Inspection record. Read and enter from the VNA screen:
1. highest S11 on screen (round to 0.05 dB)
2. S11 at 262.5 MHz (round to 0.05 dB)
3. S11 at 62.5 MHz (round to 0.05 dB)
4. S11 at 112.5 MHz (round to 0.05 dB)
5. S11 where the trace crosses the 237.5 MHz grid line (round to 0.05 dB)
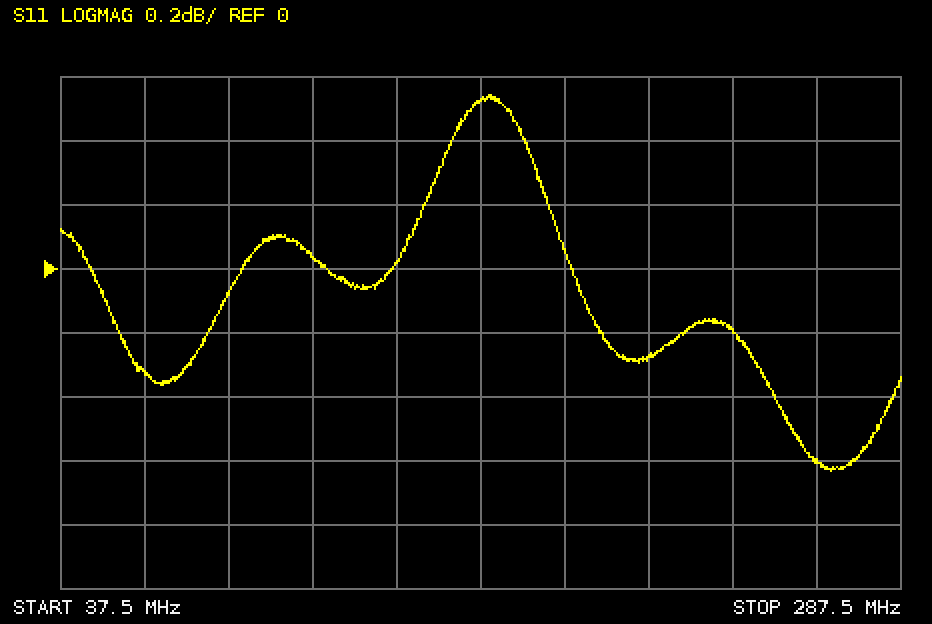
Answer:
0.55 dB
-0.60 dB
-0.30 dB
0.05 dB
-0.20 dB
